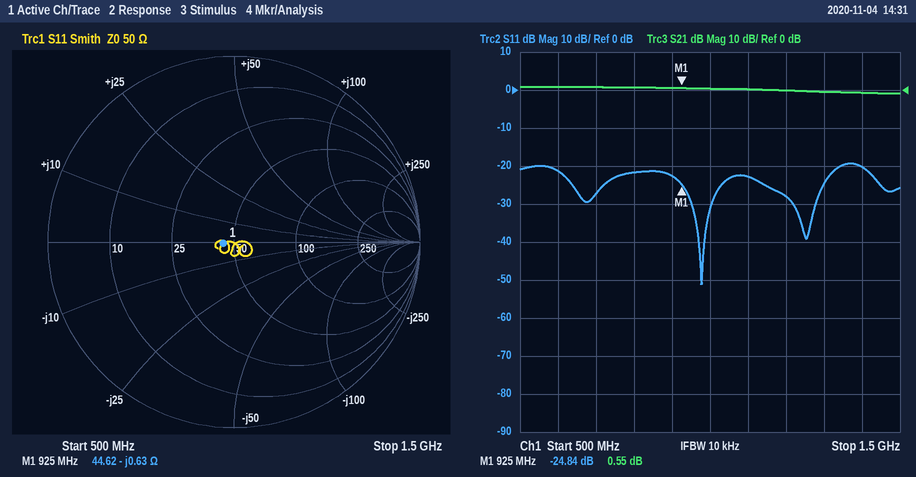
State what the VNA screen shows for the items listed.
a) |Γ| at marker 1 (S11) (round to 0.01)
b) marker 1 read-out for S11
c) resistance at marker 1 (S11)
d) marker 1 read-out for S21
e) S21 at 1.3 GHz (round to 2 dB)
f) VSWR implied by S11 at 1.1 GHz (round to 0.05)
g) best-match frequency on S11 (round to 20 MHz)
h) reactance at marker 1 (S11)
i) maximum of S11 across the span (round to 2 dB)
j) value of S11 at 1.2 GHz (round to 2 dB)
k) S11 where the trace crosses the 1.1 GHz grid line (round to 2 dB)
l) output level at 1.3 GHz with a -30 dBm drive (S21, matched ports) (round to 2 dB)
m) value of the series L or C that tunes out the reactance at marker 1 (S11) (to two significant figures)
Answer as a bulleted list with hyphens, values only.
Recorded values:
- 0.06
- -24.84 dB
- 44.62 Ω
- 0.55 dB
- 0 dB
- 1.15
- 980 MHz
- -0.63 Ω
- -20 dB
- -28 dB
- -22 dB
- -30 dBm
- 110 pH
